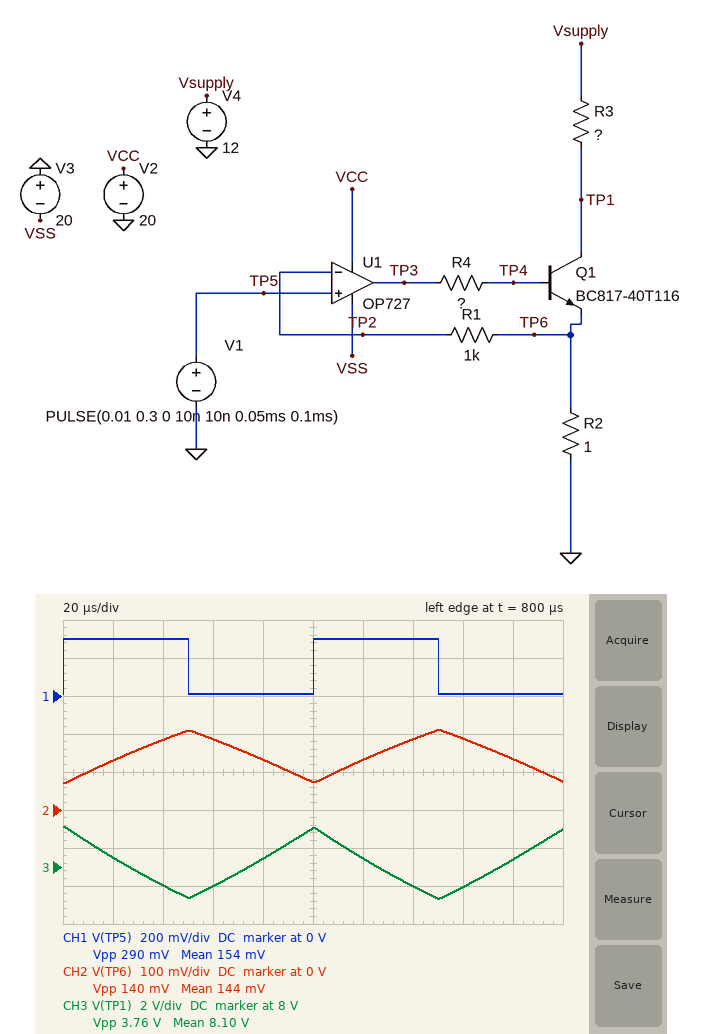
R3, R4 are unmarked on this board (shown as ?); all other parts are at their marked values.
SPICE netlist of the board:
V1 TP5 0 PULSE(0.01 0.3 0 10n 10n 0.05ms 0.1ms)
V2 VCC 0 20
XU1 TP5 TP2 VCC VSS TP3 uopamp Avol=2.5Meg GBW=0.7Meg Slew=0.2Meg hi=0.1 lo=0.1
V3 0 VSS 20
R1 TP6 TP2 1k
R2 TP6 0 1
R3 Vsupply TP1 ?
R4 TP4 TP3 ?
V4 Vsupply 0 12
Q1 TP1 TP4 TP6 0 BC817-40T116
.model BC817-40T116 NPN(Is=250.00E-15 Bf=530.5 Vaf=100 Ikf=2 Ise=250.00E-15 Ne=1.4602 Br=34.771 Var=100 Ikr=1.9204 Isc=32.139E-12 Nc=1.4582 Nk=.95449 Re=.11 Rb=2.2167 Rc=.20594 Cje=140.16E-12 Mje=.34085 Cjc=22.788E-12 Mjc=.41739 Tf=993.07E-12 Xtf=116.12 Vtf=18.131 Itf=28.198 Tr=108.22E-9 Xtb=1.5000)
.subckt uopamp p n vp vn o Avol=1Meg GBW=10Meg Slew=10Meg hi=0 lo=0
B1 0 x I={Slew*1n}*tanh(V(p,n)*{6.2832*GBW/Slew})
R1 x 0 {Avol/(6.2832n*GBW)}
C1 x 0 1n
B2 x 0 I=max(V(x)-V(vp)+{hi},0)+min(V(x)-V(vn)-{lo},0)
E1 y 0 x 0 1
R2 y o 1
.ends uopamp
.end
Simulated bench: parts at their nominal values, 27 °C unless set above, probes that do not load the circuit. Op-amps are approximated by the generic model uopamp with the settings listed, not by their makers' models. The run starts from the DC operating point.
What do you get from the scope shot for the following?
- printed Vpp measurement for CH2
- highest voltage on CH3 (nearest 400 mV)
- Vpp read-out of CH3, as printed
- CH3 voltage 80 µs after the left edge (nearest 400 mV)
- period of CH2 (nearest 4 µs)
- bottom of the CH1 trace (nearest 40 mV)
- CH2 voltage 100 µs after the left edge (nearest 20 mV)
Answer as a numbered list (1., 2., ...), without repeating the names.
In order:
1. 140 mV
2. 10.0 V
3. 3.76 V
4. 8.4 V
5. 100 µs
6. 0 V
7. 80 mV
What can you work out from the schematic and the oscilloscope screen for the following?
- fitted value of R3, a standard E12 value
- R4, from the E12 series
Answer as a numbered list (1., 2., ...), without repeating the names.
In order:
1. 27 Ω
2. 27 kΩ
